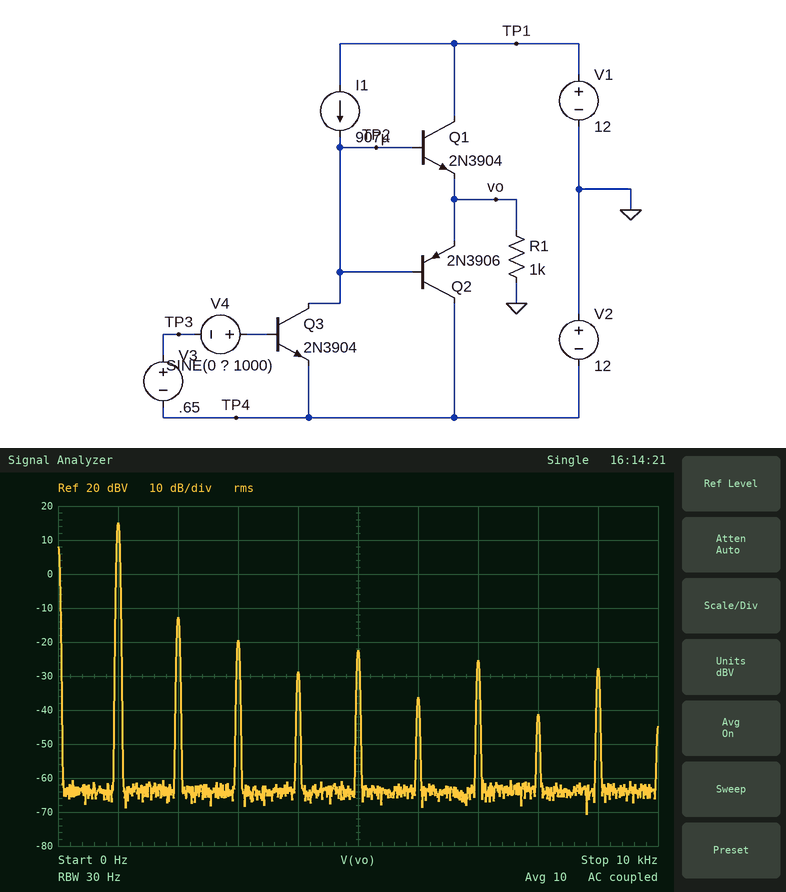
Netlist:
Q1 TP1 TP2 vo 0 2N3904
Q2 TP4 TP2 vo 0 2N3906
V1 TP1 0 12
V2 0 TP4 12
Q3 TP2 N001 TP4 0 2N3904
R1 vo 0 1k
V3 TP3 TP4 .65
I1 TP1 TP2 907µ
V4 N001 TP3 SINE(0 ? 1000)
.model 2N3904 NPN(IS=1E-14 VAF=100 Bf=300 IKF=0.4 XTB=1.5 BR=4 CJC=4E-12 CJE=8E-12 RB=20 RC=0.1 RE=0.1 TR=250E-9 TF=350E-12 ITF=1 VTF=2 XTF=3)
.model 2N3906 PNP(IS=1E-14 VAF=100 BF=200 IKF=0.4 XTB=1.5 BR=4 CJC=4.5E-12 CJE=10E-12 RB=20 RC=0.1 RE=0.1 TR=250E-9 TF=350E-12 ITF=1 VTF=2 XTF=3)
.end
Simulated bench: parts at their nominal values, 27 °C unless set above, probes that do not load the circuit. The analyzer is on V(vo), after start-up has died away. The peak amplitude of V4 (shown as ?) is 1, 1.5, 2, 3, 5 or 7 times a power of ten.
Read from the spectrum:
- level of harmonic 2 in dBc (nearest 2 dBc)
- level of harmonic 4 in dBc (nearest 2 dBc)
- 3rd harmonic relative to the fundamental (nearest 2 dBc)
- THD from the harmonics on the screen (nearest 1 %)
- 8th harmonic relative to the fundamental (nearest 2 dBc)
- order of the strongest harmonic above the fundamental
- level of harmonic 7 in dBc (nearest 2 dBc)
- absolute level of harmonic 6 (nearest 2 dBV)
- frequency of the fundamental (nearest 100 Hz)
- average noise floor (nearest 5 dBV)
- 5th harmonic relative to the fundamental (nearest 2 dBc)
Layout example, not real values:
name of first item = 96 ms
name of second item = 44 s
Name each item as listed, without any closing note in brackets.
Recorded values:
level of harmonic 2 in dBc = -28 dBc
level of harmonic 4 in dBc = -44 dBc
3rd harmonic relative to the fundamental = -34 dBc
THD from the harmonics on the screen = 5 %
8th harmonic relative to the fundamental = -56 dBc
order of the strongest harmonic above the fundamental = 2
level of harmonic 7 in dBc = -40 dBc
absolute level of harmonic 6 = -36 dBV
frequency of the fundamental = 1.0 kHz
average noise floor = -65 dBV
5th harmonic relative to the fundamental = -38 dBc
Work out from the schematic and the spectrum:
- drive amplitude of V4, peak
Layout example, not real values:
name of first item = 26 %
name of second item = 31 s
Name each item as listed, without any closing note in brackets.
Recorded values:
drive amplitude of V4, peak = 3 mV
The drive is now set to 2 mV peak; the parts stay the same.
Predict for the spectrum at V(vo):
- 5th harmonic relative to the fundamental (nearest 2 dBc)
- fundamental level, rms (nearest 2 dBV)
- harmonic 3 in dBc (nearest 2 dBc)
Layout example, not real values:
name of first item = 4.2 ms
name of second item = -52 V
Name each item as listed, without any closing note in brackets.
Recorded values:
5th harmonic relative to the fundamental = -34 dBc
fundamental level, rms = 12 dBV
harmonic 3 in dBc = -30 dBc
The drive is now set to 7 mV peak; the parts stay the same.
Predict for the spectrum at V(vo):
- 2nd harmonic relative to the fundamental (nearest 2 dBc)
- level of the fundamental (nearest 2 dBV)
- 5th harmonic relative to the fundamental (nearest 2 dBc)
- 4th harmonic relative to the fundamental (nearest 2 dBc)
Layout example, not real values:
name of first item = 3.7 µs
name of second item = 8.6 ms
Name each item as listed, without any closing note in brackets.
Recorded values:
2nd harmonic relative to the fundamental = -48 dBc
level of the fundamental = 20 dBV
5th harmonic relative to the fundamental = -60 dBc
4th harmonic relative to the fundamental = -40 dBc
